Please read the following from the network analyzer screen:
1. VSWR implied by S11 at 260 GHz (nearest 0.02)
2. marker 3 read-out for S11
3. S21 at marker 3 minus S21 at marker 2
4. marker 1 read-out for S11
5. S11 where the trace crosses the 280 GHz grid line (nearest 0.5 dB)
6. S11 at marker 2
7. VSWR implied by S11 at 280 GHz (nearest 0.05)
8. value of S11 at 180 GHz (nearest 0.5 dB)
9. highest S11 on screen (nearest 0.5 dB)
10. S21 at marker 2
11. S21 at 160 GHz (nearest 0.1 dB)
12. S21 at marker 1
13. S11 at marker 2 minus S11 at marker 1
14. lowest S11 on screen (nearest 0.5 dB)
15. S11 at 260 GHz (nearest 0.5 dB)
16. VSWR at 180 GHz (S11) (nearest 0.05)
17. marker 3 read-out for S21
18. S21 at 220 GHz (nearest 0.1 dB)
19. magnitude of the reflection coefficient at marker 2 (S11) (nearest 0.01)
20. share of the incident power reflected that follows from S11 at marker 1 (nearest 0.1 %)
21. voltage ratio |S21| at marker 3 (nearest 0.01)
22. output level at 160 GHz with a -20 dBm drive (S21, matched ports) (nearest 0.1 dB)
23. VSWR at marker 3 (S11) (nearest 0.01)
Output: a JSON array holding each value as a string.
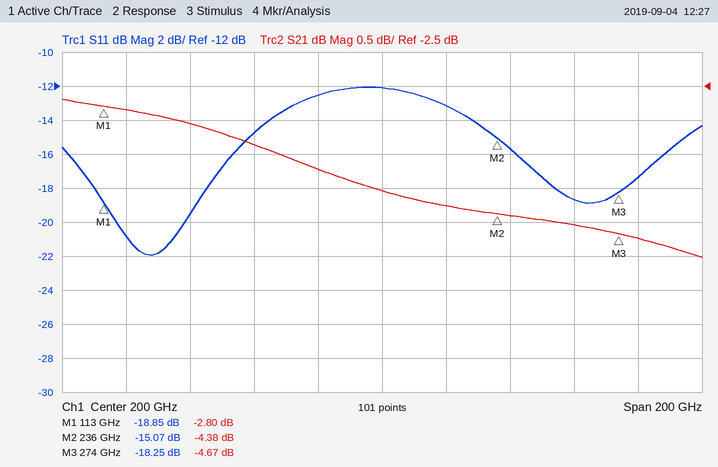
["1.26", "-18.25 dB", "-0.29 dB", "-18.85 dB", "-17.5 dB", "-15.07 dB", "1.30", "-12.5 dB", "-12.0 dB", "-4.38 dB", "-3.4 dB", "-2.80 dB", "3.78 dB", "-22.0 dB", "-18.5 dB", "1.60", "-4.67 dB", "-4.3 dB", "0.18", "1.3 %", "0.58", "-23.4 dBm", "1.28"]
